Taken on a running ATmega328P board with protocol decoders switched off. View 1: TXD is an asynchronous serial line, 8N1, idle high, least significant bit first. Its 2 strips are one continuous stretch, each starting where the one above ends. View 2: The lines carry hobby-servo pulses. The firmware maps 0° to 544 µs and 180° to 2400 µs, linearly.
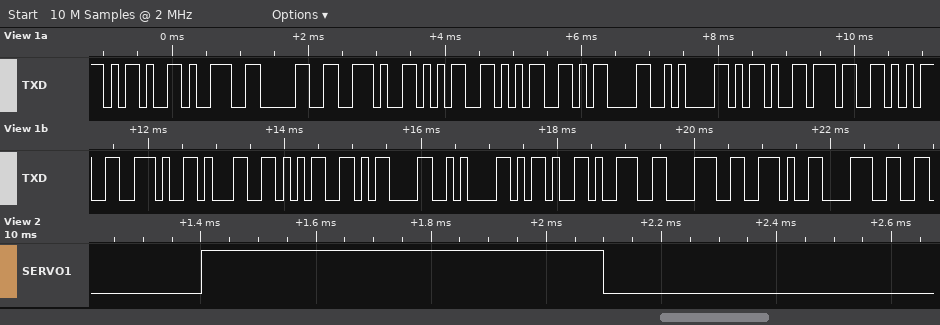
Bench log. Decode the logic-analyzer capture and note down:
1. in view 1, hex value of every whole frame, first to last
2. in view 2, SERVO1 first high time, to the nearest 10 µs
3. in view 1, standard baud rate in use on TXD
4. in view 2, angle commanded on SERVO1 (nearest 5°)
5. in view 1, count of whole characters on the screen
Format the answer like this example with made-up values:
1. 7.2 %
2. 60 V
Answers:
1. 2D 39 30 2E 35 35 0D 0A 2D 37 35 2E 31 35 0D 0A 2D 39 38 2E 38
2. 700 µs
3. 9600 baud
4. 15°
5. 21
